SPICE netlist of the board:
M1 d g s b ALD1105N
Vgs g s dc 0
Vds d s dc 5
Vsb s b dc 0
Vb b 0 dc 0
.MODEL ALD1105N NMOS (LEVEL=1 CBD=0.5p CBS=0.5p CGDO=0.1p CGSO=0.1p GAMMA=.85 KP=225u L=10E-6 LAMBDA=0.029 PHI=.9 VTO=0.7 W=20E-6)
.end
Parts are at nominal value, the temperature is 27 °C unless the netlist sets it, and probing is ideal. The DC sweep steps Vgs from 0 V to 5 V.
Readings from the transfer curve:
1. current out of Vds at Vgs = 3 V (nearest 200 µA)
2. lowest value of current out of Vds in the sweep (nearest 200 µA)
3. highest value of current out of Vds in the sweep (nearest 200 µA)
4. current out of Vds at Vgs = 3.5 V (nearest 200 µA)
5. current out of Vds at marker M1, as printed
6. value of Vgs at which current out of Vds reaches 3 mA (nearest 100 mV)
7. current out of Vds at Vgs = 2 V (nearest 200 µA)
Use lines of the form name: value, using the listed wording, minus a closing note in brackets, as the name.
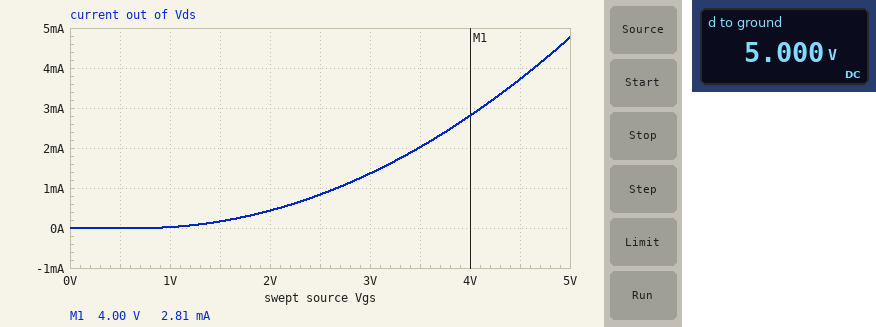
current out of Vds at Vgs = 3 V: 1.4 mA
lowest value of current out of Vds in the sweep: 0 A
highest value of current out of Vds in the sweep: 4.8 mA
current out of Vds at Vgs = 3.5 V: 2.0 mA
current out of Vds at marker M1, as printed: 2.81 mA
value of Vgs at which current out of Vds reaches 3 mA: 4.1 V
current out of Vds at Vgs = 2 V: 400 µA
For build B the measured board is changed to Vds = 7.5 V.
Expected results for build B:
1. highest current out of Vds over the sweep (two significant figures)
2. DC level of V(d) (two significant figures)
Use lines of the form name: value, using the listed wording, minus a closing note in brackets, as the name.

highest current out of Vds over the sweep: 5.1 mA
DC level of V(d): 7.5 V
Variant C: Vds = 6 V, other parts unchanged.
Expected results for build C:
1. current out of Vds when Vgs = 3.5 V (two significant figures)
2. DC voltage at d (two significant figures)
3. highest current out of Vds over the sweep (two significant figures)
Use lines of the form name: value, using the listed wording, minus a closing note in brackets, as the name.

current out of Vds when Vgs = 3.5 V: 2.1 mA
DC voltage at d: 6.0 V
highest current out of Vds over the sweep: 4.9 mA
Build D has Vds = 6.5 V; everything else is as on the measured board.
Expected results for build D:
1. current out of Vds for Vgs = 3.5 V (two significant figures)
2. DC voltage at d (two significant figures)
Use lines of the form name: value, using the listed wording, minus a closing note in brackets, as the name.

current out of Vds for Vgs = 3.5 V: 2.1 mA
DC voltage at d: 6.5 V
